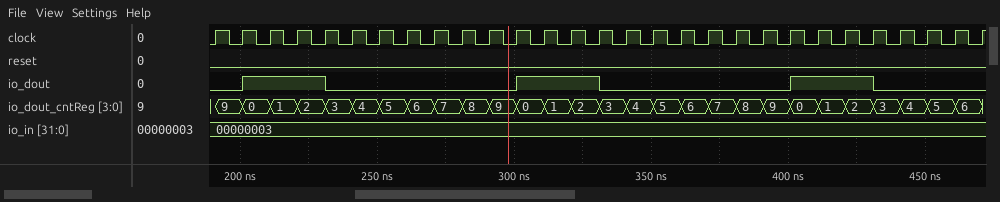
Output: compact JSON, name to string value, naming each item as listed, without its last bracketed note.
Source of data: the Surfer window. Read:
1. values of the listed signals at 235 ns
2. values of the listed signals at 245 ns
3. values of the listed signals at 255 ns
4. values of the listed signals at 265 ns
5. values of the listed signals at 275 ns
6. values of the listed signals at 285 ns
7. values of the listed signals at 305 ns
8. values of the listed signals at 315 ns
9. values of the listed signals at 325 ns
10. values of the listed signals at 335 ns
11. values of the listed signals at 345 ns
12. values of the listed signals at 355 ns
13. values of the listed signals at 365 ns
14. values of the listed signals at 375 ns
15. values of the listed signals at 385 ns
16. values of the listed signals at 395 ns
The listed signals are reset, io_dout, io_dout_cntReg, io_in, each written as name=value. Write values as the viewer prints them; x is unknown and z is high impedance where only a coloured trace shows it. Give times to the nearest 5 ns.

{"values of the listed signals at 235 ns": "reset=0, io_dout=0, io_dout_cntReg=3, io_in=00000003", "values of the listed signals at 245 ns": "reset=0, io_dout=0, io_dout_cntReg=4, io_in=00000003", "values of the listed signals at 255 ns": "reset=0, io_dout=0, io_dout_cntReg=5, io_in=00000003", "values of the listed signals at 265 ns": "reset=0, io_dout=0, io_dout_cntReg=6, io_in=00000003", "values of the listed signals at 275 ns": "reset=0, io_dout=0, io_dout_cntReg=7, io_in=00000003", "values of the listed signals at 285 ns": "reset=0, io_dout=0, io_dout_cntReg=8, io_in=00000003", "values of the listed signals at 305 ns": "reset=0, io_dout=1, io_dout_cntReg=0, io_in=00000003", "values of the listed signals at 315 ns": "reset=0, io_dout=1, io_dout_cntReg=1, io_in=00000003", "values of the listed signals at 325 ns": "reset=0, io_dout=1, io_dout_cntReg=2, io_in=00000003", "values of the listed signals at 335 ns": "reset=0, io_dout=0, io_dout_cntReg=3, io_in=00000003", "values of the listed signals at 345 ns": "reset=0, io_dout=0, io_dout_cntReg=4, io_in=00000003", "values of the listed signals at 355 ns": "reset=0, io_dout=0, io_dout_cntReg=5, io_in=00000003", "values of the listed signals at 365 ns": "reset=0, io_dout=0, io_dout_cntReg=6, io_in=00000003", "values of the listed signals at 375 ns": "reset=0, io_dout=0, io_dout_cntReg=7, io_in=00000003", "values of the listed signals at 385 ns": "reset=0, io_dout=0, io_dout_cntReg=8, io_in=00000003", "values of the listed signals at 395 ns": "reset=0, io_dout=0, io_dout_cntReg=9, io_in=00000003"}
